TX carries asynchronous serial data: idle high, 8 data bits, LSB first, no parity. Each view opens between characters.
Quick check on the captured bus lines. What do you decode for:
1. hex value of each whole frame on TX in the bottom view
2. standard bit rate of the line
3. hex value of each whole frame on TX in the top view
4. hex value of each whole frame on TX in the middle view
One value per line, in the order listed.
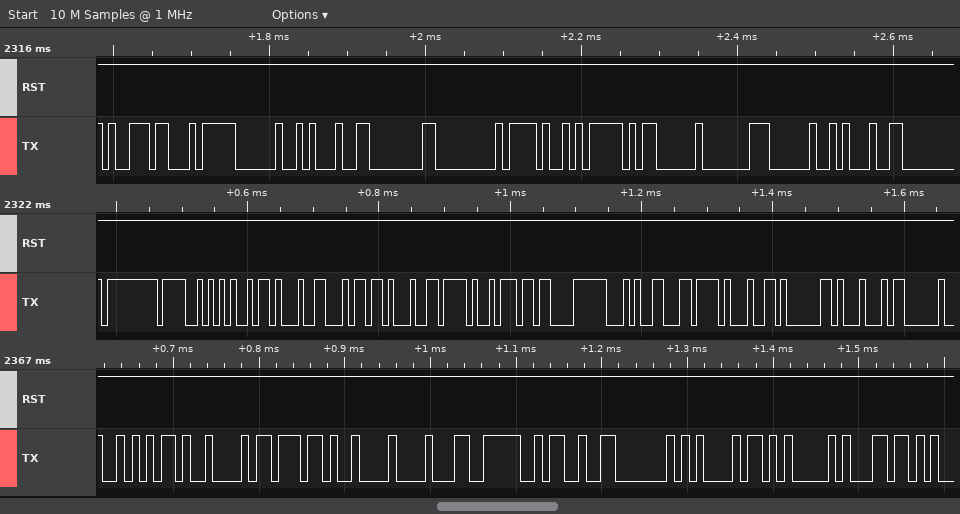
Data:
AA, 09, BB, 09, 88, 3E, 93, 40, A1, 05, B1
115200 baud
B9, F4, 20, 91, 80, 00, 2F, 7D, 03, C0, 20, 91
FF, 4F, A5, 91, B4, 91, 2F, B7, F8, 94, EC, 91, 81, 11, 03
